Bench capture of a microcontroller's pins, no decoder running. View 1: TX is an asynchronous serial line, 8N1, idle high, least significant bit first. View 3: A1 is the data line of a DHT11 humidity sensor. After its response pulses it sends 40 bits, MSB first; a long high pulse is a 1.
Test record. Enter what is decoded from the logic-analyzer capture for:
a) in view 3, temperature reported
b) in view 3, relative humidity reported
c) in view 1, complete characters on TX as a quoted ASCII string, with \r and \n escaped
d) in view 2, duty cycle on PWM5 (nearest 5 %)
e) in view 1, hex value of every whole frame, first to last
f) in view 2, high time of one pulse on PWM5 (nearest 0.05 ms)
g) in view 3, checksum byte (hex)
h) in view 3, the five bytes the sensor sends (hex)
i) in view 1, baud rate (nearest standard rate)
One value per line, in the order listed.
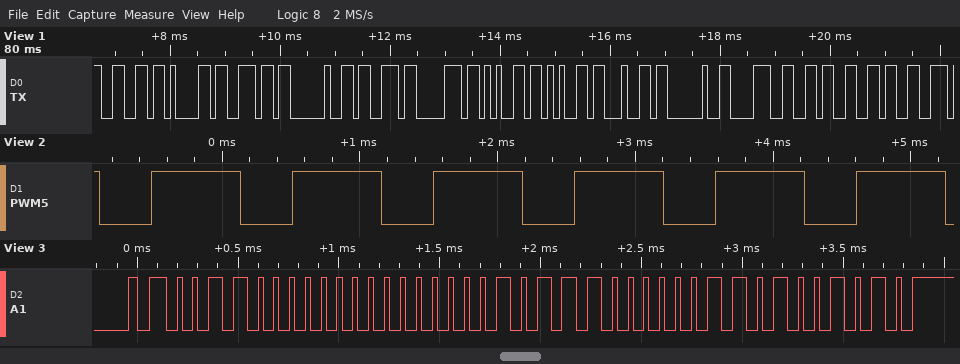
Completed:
23.3 °C
48 %
"fan speed 866"
65 %
66 61 6E 20 73 70 65 65 64 20 38 36 36
0.65 ms
0x4A
30 00 17 03 4A
9600 baud
